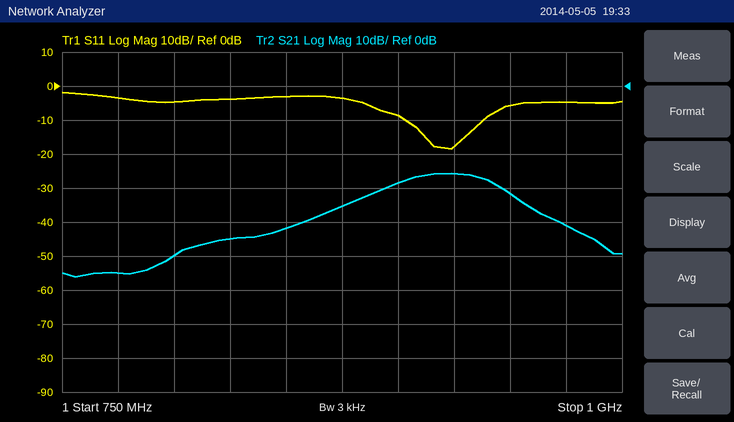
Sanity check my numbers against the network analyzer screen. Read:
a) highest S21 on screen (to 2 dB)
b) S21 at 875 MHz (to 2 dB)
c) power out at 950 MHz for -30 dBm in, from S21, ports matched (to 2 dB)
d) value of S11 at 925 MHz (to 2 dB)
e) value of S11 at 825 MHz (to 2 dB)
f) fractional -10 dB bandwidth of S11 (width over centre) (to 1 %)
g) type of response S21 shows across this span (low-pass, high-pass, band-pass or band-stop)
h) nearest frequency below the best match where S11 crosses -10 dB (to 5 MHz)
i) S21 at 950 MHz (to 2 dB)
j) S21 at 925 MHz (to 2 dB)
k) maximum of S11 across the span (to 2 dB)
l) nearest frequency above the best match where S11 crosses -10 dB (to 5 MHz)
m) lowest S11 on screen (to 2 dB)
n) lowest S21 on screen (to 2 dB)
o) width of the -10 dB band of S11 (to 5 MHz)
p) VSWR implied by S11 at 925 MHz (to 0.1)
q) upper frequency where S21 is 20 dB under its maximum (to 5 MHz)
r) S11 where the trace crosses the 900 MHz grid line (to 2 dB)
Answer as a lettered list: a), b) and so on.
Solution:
a) -26 dB
b) -36 dB
c) -62 dBm
d) -18 dB
e) -4 dB
f) 4 %
g) band-pass
h) 905 MHz
i) -32 dB
j) -26 dB
k) -2 dB
l) 940 MHz
m) -18 dB
n) -56 dB
o) 35 MHz
p) 1.3
q) 990 MHz
r) -8 dB
